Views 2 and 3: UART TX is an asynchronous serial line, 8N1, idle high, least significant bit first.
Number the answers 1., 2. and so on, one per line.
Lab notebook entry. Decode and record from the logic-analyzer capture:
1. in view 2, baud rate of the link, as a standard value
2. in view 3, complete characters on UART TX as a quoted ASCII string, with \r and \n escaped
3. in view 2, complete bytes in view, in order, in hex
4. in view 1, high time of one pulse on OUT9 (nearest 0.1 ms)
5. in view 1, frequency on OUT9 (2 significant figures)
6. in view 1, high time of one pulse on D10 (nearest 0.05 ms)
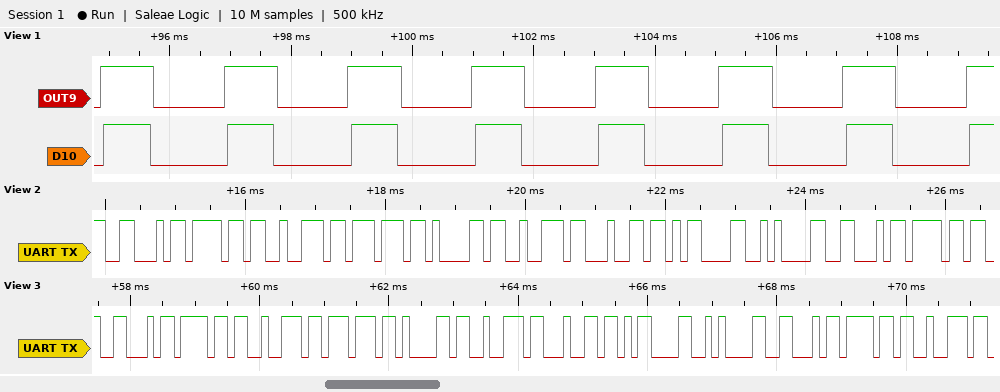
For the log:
1. 9600 baud
2. "Forward\r\nFor"
3. 46 6F 72 77 61 72 64 0D 0A 46 6F
4. 0.9 ms
5. 490 Hz
6. 0.75 ms
